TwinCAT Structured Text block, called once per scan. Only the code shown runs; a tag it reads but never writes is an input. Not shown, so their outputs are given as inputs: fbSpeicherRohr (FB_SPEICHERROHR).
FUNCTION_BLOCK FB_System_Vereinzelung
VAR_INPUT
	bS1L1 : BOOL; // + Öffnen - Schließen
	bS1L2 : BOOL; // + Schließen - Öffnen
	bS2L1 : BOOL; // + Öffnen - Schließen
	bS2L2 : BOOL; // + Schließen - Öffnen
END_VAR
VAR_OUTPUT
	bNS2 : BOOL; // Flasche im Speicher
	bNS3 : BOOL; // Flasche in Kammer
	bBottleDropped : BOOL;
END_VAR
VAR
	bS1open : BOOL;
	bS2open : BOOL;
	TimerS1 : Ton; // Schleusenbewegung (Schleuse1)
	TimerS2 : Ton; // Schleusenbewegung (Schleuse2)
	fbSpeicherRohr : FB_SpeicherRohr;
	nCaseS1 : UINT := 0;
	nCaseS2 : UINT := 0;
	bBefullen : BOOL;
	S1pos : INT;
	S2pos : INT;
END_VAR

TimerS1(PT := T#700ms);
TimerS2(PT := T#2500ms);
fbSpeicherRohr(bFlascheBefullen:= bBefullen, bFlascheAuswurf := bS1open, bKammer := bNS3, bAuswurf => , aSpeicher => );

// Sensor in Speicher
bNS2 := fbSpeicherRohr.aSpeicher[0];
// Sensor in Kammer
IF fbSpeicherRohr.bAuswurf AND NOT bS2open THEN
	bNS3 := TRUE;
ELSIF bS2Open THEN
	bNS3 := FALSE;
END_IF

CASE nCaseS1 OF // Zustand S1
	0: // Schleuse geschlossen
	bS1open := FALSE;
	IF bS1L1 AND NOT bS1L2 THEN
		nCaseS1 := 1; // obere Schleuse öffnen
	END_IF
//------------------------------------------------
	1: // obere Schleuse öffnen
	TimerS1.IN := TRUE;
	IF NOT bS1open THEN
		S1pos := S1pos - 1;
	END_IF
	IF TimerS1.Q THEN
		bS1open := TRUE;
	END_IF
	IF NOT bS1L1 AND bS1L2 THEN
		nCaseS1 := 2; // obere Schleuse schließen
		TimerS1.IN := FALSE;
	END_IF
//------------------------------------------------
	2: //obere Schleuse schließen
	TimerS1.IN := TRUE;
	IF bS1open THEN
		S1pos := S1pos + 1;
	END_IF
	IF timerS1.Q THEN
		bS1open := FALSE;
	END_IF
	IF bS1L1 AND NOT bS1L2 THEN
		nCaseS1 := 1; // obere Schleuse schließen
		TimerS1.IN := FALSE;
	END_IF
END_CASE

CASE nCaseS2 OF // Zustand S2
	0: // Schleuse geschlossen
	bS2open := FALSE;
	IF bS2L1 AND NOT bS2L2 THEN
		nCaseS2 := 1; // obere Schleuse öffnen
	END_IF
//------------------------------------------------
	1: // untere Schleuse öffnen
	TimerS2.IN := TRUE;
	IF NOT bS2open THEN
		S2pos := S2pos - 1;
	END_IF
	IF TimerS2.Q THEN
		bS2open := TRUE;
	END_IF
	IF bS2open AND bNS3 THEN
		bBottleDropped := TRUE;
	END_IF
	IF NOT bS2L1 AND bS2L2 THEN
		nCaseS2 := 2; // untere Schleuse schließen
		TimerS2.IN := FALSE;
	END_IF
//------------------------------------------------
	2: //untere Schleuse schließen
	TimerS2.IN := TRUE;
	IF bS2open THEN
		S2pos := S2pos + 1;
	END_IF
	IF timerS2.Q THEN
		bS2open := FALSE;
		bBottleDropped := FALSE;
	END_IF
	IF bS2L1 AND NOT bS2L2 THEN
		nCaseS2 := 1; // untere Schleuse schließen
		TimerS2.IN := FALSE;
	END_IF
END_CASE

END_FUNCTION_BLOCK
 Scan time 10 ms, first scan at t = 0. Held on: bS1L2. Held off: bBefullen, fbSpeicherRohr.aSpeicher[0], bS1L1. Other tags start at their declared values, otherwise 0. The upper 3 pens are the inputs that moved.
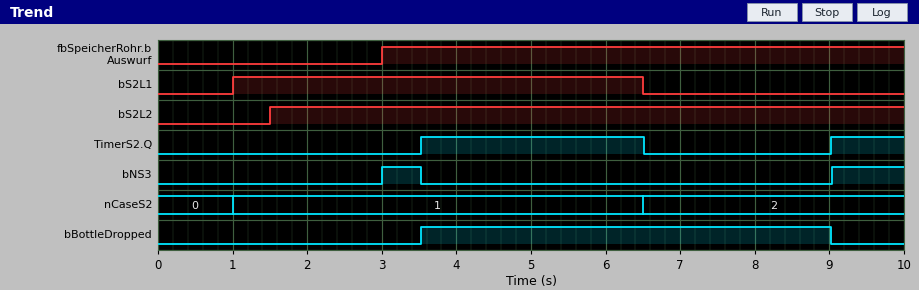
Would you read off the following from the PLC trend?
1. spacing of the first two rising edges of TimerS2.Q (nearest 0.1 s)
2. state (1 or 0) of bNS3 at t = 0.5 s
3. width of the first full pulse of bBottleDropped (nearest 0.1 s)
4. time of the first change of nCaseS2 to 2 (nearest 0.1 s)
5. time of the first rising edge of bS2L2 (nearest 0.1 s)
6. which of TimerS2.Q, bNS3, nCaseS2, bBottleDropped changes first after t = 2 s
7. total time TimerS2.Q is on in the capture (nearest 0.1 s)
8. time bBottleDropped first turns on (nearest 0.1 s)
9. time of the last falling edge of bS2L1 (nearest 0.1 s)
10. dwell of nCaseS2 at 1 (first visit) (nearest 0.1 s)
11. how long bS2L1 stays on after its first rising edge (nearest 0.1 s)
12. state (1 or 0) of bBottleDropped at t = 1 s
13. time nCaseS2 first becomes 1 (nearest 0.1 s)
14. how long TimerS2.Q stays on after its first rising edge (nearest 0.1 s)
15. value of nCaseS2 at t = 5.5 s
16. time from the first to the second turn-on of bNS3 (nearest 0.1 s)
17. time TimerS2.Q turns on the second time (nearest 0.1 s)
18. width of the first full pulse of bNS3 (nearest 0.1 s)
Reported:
5.5 s
0
5.5 s
6.5 s
1.5 s
bNS3
4.0 s
3.5 s
6.5 s
5.5 s
5.5 s
0
1.0 s
3.0 s
1
6.0 s
9.0 s
0.5 s
